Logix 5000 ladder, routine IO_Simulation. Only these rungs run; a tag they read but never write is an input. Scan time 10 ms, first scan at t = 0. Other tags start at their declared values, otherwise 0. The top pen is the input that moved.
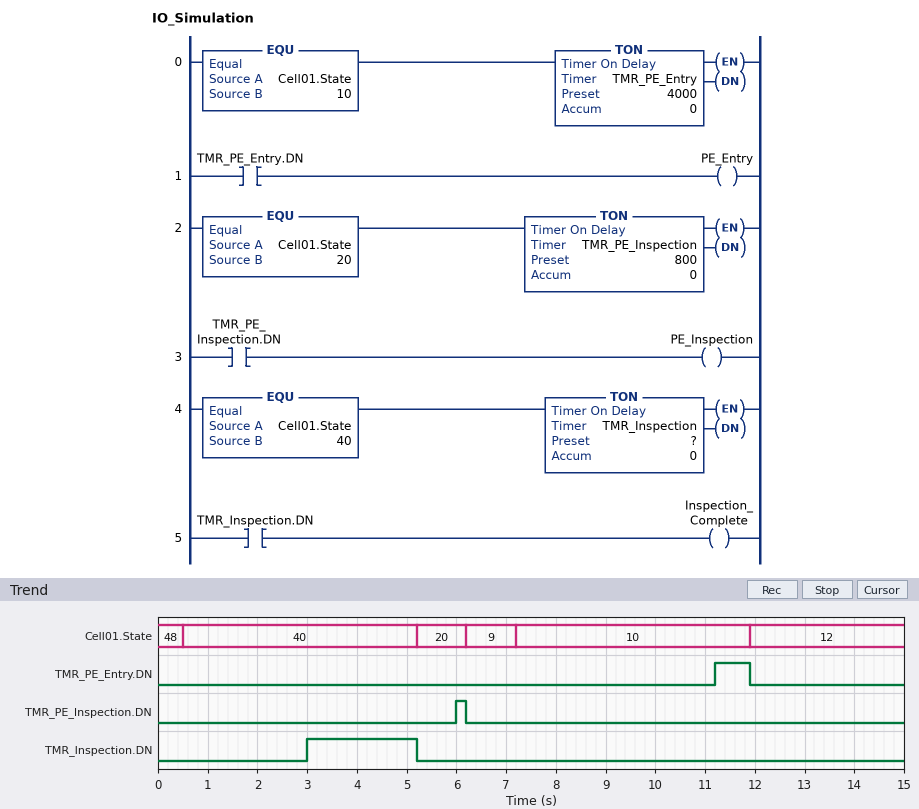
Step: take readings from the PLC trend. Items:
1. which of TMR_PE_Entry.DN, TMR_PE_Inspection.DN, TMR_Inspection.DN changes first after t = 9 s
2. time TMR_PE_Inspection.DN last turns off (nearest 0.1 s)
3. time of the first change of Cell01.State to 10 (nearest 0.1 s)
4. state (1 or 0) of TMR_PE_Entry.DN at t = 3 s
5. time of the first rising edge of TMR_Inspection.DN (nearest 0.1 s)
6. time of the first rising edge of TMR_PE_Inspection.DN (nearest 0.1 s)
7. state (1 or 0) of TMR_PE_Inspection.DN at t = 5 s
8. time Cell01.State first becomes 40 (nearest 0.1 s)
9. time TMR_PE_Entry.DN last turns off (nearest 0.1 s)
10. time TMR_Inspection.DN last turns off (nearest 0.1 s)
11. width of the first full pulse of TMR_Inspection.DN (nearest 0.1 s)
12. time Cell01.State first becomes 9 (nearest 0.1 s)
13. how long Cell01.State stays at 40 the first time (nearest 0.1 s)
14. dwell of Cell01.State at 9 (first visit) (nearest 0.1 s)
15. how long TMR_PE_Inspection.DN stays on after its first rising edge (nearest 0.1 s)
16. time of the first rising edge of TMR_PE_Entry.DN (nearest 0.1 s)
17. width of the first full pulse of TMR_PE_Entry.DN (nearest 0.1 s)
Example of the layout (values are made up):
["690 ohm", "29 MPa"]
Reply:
["TMR_PE_Entry.DN", "6.2 s", "7.2 s", "0", "3.0 s", "6.0 s", "0", "0.5 s", "11.9 s", "5.2 s", "2.2 s", "6.2 s", "4.7 s", "1.0 s", "0.2 s", "11.2 s", "0.7 s"]
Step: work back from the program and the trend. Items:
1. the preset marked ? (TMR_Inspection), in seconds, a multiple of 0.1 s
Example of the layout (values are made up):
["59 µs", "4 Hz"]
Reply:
["2.5 s"]
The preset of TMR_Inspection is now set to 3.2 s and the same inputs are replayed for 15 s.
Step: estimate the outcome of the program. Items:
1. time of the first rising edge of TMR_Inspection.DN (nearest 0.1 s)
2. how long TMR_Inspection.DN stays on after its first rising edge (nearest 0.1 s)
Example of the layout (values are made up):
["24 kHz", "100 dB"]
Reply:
["3.7 s", "1.5 s"]
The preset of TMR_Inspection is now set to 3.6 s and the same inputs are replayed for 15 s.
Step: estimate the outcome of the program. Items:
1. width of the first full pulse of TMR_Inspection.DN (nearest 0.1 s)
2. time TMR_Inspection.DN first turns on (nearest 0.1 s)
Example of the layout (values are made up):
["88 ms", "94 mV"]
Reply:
["1.1 s", "4.1 s"]
